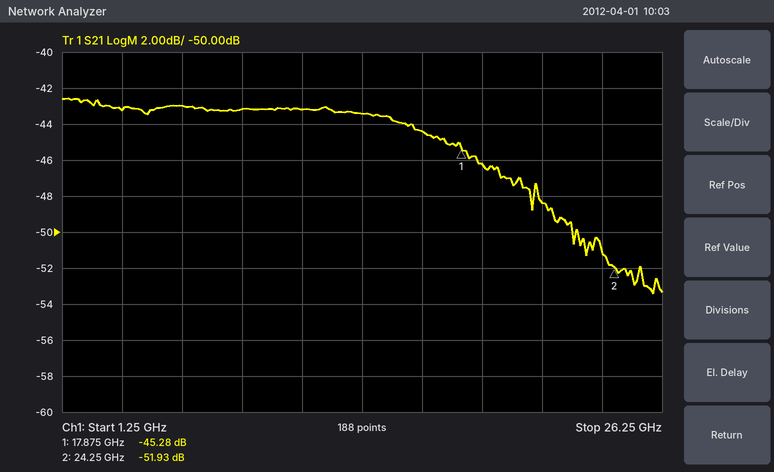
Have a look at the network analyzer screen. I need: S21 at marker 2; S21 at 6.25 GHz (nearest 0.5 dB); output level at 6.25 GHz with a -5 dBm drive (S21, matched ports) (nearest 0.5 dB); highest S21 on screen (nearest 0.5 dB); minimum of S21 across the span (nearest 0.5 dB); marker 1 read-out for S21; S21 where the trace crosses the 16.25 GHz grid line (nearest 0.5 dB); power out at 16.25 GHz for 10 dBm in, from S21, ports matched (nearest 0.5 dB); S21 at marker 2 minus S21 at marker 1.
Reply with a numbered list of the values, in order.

1. -51.93 dB
2. -43.0 dB
3. -48.0 dBm
4. -42.5 dB
5. -53.5 dB
6. -45.28 dB
7. -44.5 dB
8. -34.5 dBm
9. -6.65 dB
